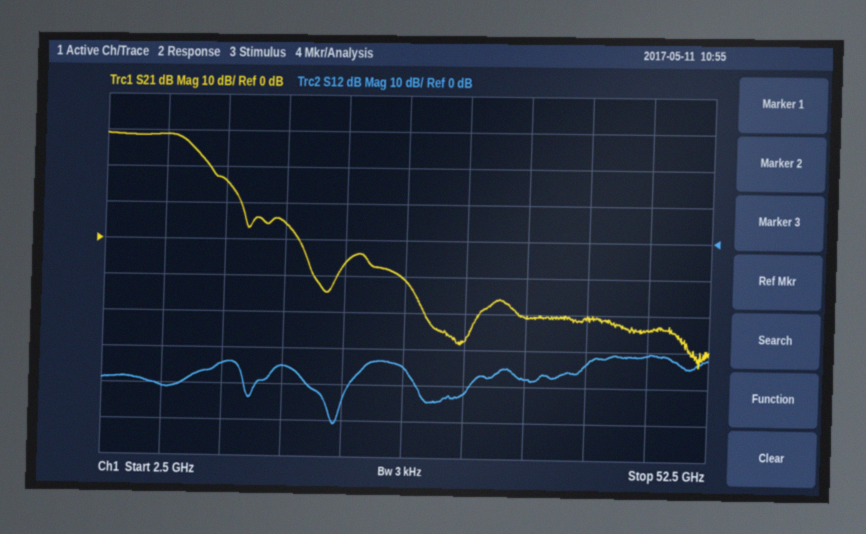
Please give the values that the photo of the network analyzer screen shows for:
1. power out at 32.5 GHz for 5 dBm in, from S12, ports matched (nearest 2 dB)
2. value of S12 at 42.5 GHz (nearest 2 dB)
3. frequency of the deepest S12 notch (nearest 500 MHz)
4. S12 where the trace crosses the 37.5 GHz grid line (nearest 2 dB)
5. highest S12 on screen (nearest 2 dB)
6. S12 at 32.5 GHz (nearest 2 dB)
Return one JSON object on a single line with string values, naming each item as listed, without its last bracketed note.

{"power out at 32.5 GHz for 5 dBm in, from S12, ports matched": "-38 dBm", "value of S12 at 42.5 GHz": "-34 dB", "frequency of the deepest S12 notch": "22.0 GHz", "S12 where the trace crosses the 37.5 GHz grid line": "-38 dB", "highest S12 on screen": "-30 dB", "S12 at 32.5 GHz": "-42 dB"}
